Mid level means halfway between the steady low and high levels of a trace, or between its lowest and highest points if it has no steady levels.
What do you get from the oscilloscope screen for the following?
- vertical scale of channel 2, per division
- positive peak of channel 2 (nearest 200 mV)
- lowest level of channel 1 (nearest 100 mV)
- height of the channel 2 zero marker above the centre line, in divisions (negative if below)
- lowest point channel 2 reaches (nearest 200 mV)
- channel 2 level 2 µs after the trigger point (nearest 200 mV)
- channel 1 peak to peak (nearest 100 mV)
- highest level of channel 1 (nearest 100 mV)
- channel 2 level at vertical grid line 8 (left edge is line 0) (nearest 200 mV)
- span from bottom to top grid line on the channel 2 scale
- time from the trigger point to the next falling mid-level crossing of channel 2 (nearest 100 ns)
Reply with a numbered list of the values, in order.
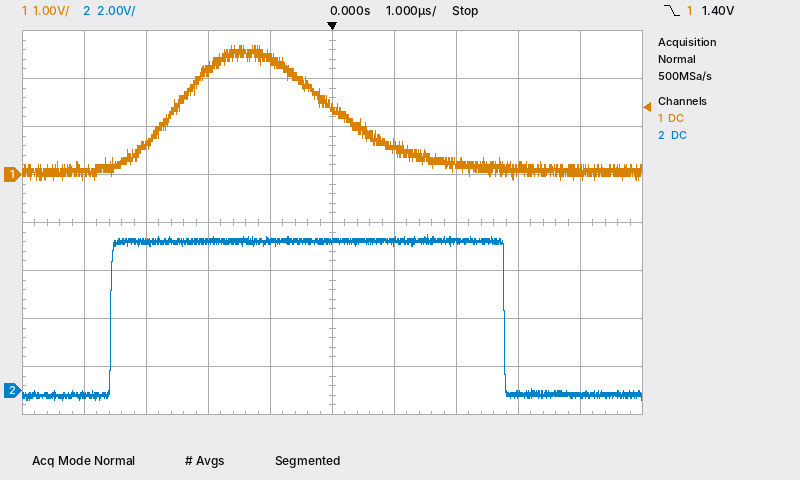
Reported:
1. 2 V
2. 6.4 V
3. -100 mV
4. -3.5 div
5. -400 mV
6. 6.2 V
7. 2.8 V
8. 2.7 V
9. -200 mV
10. 16 V
11. 2.8 µs
